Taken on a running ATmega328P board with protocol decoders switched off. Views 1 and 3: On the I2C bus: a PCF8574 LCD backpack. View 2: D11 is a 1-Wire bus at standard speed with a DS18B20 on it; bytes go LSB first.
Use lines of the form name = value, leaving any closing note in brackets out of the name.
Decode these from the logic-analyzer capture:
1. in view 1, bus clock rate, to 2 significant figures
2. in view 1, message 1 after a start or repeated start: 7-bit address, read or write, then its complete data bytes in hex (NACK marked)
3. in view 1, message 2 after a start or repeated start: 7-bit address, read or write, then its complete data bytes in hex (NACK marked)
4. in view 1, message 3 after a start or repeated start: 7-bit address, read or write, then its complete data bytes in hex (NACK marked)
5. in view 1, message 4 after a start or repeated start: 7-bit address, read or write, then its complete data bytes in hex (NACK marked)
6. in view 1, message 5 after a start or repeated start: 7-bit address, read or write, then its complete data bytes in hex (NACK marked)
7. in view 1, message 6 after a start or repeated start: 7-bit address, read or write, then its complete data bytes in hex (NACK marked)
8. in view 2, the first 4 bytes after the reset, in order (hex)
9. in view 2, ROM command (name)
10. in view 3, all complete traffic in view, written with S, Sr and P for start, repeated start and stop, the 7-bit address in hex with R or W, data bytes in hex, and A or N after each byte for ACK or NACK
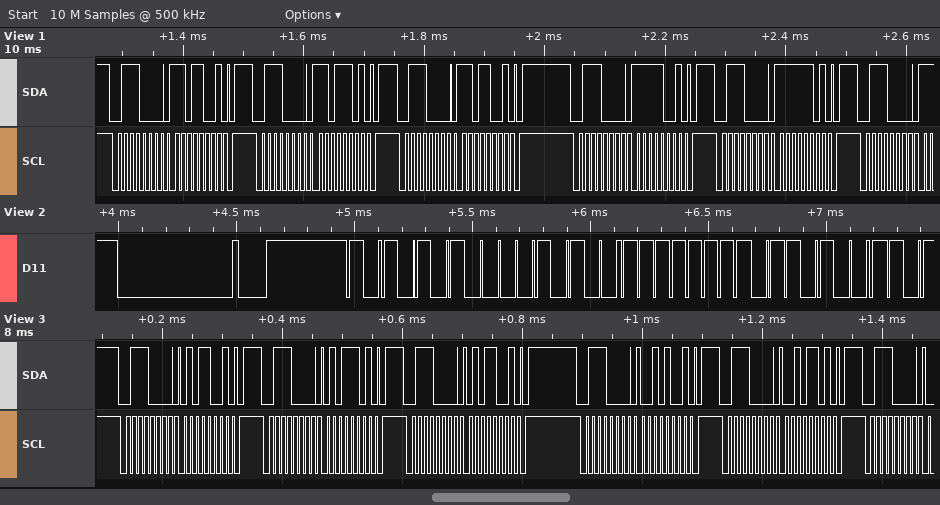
in view 1, bus clock rate, to 2 significant figures = 100 kHz
in view 1, message 1 after a start or repeated start: 7-bit address, read or write, then its complete data bytes in hex = 0x38 write: D9
in view 1, message 2 after a start or repeated start: 7-bit address, read or write, then its complete data bytes in hex = 0x38 write: DD
in view 1, message 3 after a start or repeated start: 7-bit address, read or write, then its complete data bytes in hex = 0x38 write: D9
in view 1, message 4 after a start or repeated start: 7-bit address, read or write, then its complete data bytes in hex = 0x38 write: F9
in view 1, message 5 after a start or repeated start: 7-bit address, read or write, then its complete data bytes in hex = 0x38 write: FD
in view 1, message 6 after a start or repeated start: 7-bit address, read or write, then its complete data bytes in hex = 0x38 write
in view 2, the first 4 bytes after the reset, in order = 55 28 FF 96
in view 2, ROM command = Match ROM
in view 3, all complete traffic in view, written with S, Sr and P for start, repeated start and stop, the 7-bit address in hex with R or W, data bytes in hex, and A or N after each byte for ACK or NACK = S 38W A 59 A P S 38W A 5D A P S 38W A 59 A P S 38W A 29 A P S 38W A 2D A P S 38W A
